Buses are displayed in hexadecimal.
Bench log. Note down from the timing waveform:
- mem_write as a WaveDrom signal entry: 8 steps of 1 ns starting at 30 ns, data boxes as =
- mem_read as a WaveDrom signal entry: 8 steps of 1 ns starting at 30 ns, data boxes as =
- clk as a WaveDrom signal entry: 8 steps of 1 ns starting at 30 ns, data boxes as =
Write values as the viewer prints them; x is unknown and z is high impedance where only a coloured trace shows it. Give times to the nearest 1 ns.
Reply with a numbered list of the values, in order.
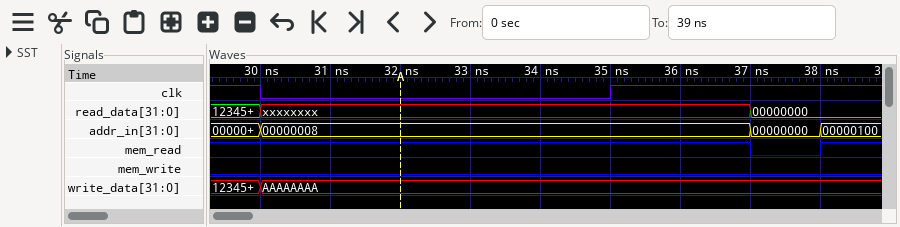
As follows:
1. {name: 'mem_write', wave: '0.......'}
2. {name: 'mem_read', wave: '1......0'}
3. {name: 'clk', wave: '0....1..'}
